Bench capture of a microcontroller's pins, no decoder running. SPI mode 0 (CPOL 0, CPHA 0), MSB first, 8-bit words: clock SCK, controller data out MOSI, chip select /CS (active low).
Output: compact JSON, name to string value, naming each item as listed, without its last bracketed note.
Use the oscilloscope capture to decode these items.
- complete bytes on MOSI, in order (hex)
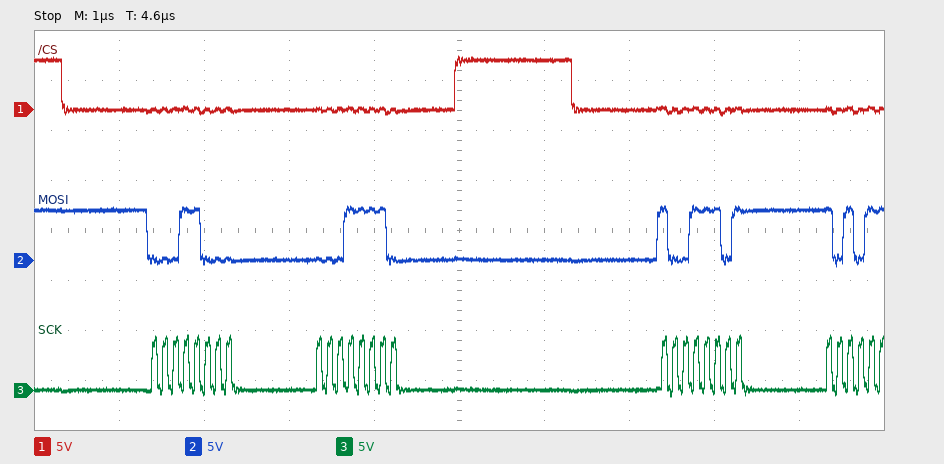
{"complete bytes on MOSI, in order": "18 1E 9D"}
